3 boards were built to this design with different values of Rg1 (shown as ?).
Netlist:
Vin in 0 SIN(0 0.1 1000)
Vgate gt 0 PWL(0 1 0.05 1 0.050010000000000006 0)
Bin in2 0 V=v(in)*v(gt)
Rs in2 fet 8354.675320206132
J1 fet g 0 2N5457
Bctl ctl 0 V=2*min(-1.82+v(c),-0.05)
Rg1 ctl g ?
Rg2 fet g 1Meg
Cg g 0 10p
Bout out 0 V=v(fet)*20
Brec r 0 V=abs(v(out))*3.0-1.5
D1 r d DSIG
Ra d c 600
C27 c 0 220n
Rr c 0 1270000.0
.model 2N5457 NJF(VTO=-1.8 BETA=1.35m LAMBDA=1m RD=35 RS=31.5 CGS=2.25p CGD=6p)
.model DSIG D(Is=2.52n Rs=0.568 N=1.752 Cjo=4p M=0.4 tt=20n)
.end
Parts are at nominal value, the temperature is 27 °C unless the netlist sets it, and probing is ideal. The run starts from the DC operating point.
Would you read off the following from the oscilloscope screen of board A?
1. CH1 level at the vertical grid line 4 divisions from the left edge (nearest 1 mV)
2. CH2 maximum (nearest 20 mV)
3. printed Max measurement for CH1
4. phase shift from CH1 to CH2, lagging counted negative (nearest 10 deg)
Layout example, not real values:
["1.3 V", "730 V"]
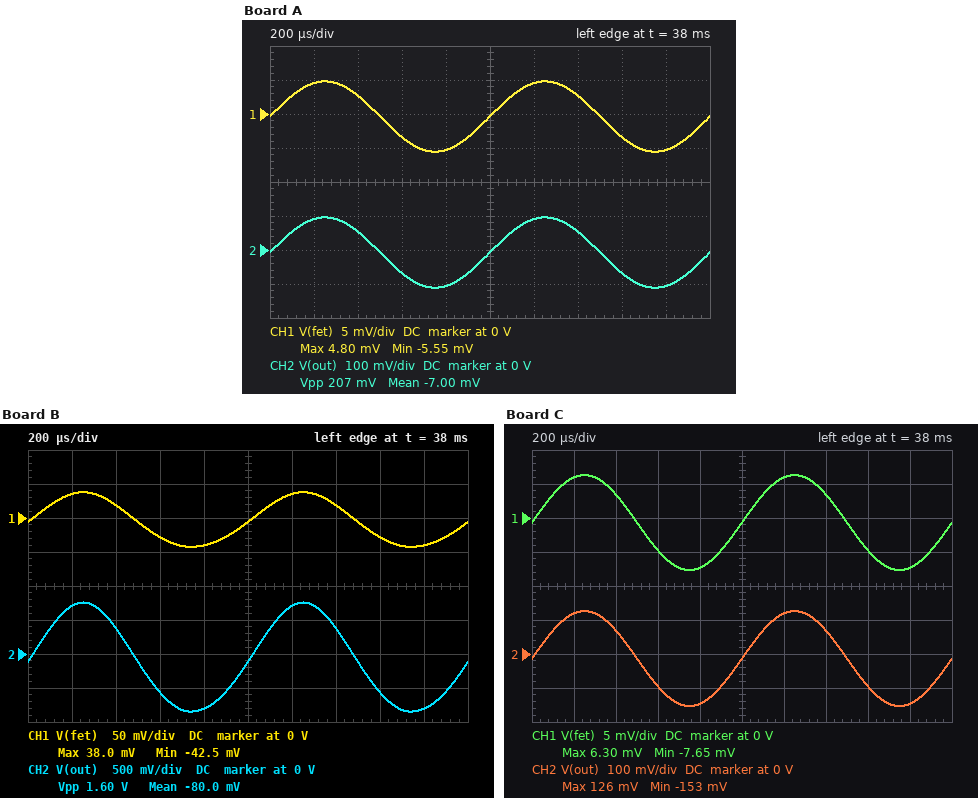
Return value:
["-5 mV", "100 mV", "4.80 mV", "0 deg"]
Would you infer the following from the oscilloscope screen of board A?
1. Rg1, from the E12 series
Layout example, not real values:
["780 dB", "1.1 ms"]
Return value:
["3.3 MΩ"]
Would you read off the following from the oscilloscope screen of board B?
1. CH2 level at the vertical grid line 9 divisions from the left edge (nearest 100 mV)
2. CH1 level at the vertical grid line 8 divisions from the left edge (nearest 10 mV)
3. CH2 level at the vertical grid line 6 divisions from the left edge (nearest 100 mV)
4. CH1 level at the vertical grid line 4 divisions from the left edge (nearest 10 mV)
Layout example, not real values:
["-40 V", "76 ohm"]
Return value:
["-800 mV", "-30 mV", "700 mV", "-40 mV"]
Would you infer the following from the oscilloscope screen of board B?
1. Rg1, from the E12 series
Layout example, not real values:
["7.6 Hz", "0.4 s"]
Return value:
["330 kΩ"]
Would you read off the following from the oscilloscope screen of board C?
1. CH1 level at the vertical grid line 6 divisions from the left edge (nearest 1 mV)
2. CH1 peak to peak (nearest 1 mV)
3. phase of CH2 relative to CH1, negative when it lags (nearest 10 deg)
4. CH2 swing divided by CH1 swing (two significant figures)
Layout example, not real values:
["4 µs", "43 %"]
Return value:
["6 mV", "14 mV", "0 deg", "20"]
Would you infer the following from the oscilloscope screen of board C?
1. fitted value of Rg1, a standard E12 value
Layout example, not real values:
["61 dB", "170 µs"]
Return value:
["2.2 MΩ"]
